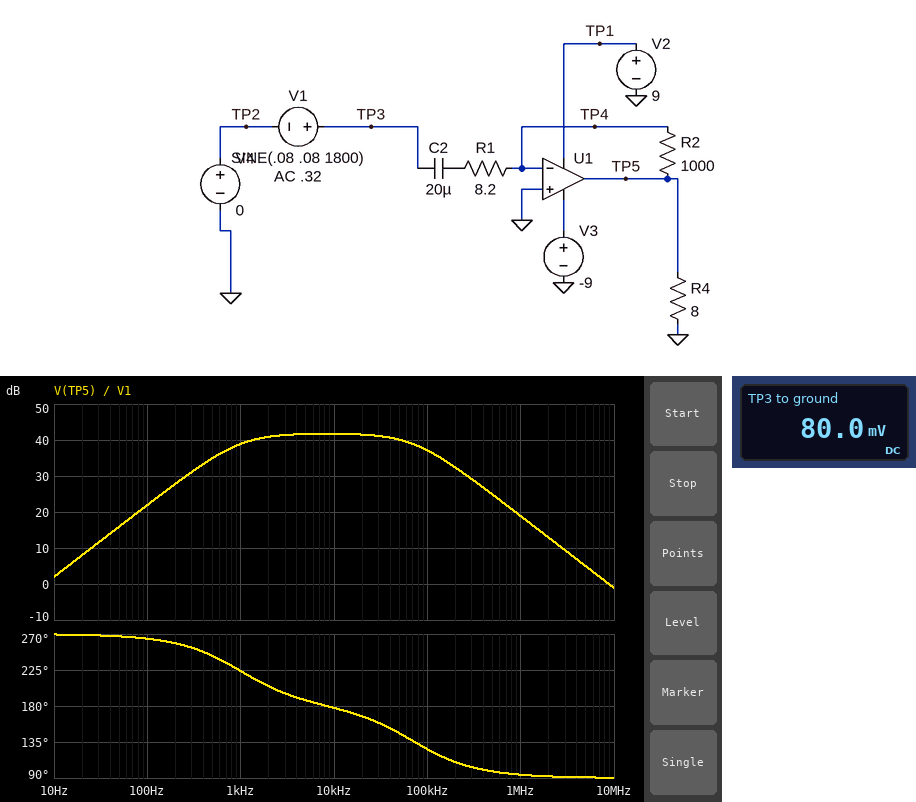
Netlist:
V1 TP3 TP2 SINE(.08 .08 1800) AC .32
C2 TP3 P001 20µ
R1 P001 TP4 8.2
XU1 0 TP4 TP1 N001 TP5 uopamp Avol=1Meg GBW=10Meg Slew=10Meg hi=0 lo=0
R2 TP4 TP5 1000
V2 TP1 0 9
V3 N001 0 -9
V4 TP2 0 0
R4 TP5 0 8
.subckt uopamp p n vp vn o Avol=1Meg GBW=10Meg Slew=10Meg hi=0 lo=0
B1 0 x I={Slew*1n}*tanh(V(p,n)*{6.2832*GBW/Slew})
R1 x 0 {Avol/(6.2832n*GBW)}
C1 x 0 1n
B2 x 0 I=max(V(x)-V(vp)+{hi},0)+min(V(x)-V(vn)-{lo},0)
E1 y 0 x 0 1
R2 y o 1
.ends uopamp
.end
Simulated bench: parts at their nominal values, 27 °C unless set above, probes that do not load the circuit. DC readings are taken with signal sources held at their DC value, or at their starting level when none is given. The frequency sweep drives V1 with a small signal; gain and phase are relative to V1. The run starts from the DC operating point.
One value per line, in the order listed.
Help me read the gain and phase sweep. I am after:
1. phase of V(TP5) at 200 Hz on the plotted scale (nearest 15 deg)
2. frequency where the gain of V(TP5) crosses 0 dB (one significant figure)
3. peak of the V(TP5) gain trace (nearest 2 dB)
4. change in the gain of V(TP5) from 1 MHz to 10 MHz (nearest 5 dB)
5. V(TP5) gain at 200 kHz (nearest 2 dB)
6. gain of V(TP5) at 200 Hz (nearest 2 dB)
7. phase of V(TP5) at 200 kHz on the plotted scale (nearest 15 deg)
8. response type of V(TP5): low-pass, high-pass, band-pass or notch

255 deg
9 MHz
42 dB
-20 dB
32 dB
28 dB
105 deg
band-pass
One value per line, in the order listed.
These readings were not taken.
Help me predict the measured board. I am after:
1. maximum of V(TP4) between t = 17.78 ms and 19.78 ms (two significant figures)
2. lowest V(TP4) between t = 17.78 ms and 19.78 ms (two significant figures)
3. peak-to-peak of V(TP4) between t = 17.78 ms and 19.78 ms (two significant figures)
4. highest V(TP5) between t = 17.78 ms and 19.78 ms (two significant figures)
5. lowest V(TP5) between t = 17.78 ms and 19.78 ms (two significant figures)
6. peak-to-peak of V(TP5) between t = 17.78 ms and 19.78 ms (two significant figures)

6.0 mV
-6.0 mV
12 mV
8.0 V
-8.0 V
16 V
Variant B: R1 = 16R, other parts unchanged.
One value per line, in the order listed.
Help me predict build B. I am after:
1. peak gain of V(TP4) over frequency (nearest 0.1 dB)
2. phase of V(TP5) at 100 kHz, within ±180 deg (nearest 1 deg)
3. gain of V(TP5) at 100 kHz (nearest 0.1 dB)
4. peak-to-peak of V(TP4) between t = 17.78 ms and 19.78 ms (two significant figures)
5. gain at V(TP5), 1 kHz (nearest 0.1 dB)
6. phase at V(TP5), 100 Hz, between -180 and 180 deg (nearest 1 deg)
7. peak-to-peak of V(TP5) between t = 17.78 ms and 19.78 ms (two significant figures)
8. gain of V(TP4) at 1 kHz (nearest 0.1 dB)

-0.1 dB
145 deg
34.1 dB
2.0 mV
35.0 dB
-101 deg
9.7 V
-44.0 dB
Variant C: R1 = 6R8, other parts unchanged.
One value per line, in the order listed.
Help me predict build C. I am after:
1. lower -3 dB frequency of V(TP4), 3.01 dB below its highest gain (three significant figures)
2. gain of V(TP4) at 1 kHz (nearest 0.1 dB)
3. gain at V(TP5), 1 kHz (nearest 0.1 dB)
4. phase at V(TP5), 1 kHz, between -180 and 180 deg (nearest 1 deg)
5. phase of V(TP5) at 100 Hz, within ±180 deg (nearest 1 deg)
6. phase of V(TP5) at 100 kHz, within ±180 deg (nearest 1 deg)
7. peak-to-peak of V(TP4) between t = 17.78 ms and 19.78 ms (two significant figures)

58.8 kHz
-39.3 dB
39.7 dB
-131 deg
-95 deg
121 deg
32 mV
